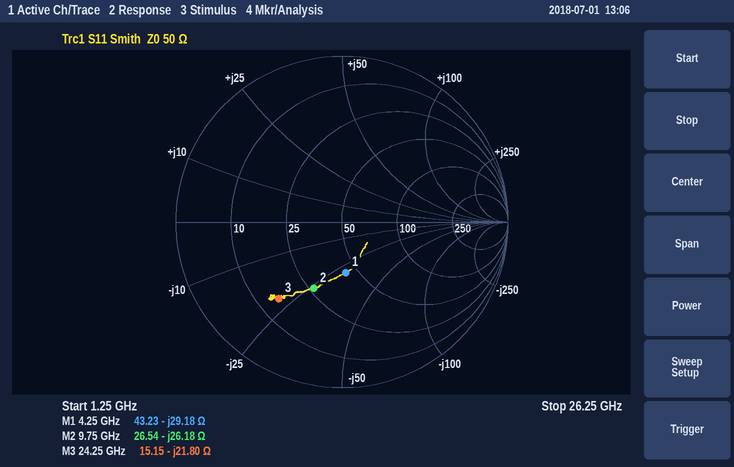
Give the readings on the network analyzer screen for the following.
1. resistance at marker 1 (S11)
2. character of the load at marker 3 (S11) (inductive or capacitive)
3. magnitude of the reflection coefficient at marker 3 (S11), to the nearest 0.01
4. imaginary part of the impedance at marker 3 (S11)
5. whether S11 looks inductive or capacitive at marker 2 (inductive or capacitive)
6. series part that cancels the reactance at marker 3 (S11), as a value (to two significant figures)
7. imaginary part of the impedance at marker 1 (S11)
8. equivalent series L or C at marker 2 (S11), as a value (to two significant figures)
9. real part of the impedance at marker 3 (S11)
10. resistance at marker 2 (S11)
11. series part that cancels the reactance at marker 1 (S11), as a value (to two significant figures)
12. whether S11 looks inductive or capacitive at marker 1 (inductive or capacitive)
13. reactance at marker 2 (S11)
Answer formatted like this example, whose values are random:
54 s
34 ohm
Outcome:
43.23 Ω
capacitive
0.60
-21.80 Ω
capacitive
140 pH
-29.18 Ω
620 fF
15.15 Ω
26.54 Ω
1.1 nH
capacitive
-26.18 Ω
